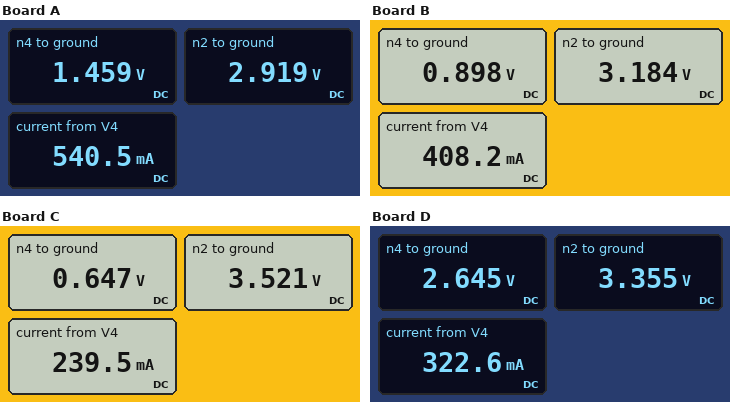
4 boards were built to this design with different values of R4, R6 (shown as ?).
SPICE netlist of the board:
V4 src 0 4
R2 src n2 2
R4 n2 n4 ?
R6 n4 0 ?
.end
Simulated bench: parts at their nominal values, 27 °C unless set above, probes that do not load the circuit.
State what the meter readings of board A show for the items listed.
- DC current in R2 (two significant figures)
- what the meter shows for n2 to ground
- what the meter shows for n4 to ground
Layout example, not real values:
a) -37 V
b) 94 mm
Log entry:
a) 540 mA
b) 2.919 V
c) 1.459 V
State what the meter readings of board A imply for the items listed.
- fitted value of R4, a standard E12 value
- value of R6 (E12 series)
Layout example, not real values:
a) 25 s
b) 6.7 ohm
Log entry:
a) 2.7 Ω
b) 2.7 Ω
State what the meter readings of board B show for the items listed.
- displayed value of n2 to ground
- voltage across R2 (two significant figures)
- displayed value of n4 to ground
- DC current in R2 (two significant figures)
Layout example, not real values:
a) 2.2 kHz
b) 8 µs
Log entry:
a) 3.184 V
b) 820 mV
c) 0.898 V
d) 410 mA
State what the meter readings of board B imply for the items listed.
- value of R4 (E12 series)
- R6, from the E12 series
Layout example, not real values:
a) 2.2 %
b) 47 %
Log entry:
a) 5.6 Ω
b) 2.2 Ω
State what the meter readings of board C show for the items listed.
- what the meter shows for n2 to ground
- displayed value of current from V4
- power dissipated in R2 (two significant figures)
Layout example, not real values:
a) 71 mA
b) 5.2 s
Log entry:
a) 3.521 V
b) 239.5 mA
c) 110 mW
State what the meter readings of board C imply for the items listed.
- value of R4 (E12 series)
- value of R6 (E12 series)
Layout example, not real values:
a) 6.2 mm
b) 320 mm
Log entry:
a) 12 Ω
b) 2.7 Ω
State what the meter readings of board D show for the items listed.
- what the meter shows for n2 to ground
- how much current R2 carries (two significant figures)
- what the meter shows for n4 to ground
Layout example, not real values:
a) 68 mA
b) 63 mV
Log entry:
a) 3.355 V
b) 320 mA
c) 2.645 V
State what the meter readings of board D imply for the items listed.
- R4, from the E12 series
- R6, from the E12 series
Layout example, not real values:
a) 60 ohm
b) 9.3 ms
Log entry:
a) 2.2 Ω
b) 8.2 Ω
